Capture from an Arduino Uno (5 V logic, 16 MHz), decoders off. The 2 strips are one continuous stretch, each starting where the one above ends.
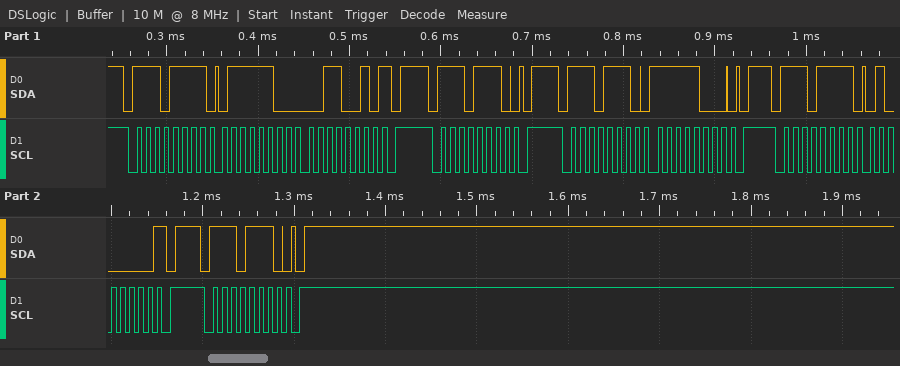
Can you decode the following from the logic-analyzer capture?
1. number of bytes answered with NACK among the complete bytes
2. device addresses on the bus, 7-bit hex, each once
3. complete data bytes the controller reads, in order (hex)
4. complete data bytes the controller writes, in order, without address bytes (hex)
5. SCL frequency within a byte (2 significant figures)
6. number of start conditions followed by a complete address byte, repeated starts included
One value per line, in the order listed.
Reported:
2
0x77
7C 32 40
F8
100 kHz
5
